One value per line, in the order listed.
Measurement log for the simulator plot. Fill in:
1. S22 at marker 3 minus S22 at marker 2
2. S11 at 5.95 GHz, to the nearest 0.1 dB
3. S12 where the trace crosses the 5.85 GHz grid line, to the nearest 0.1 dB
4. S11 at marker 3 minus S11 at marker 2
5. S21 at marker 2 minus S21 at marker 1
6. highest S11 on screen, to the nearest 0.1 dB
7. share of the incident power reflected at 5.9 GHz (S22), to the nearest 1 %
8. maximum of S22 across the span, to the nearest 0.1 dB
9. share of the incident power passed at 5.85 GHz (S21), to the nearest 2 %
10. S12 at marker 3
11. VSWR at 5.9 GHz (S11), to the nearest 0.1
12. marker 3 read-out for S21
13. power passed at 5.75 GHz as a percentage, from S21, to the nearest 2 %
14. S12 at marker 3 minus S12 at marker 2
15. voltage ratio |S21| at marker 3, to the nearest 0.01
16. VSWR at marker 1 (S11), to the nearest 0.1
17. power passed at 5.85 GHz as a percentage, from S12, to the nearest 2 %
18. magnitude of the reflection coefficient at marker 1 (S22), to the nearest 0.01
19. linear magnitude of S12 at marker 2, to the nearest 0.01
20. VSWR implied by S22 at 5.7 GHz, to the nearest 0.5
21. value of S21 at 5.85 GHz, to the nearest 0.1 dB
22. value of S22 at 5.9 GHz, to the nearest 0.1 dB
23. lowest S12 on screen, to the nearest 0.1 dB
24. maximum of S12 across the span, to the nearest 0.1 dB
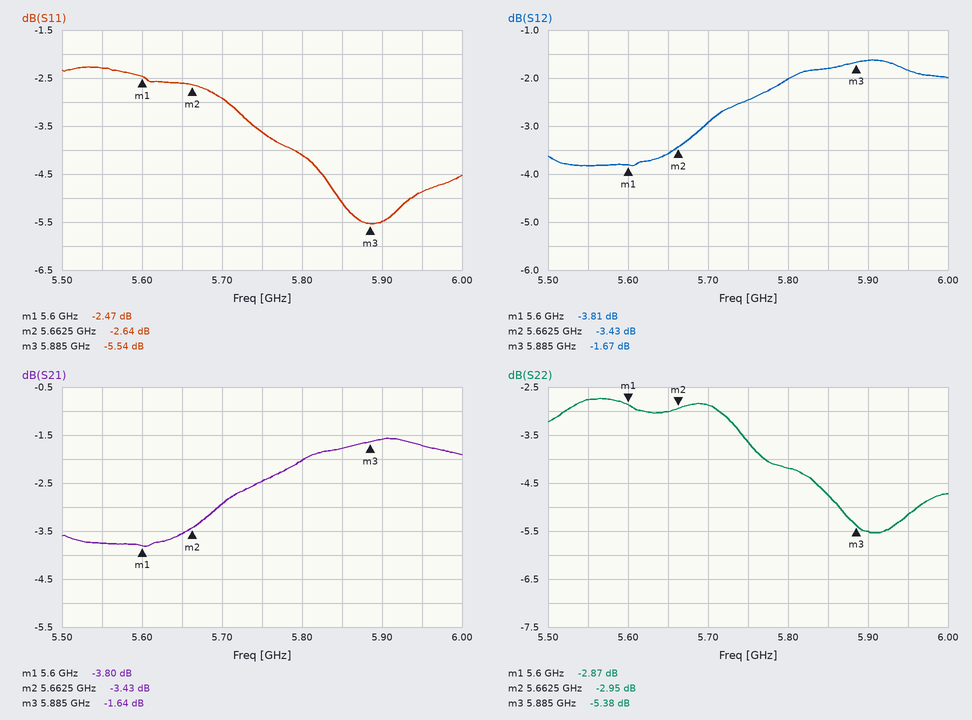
-2.43 dB
-4.9 dB
-1.8 dB
-2.90 dB
0.37 dB
-2.3 dB
28 %
-2.7 dB
66 %
-1.67 dB
3.3
-1.64 dB
56 %
1.76 dB
0.83
7.1
66 %
0.72
0.67
6.0
-1.8 dB
-5.5 dB
-3.8 dB
-1.6 dB
